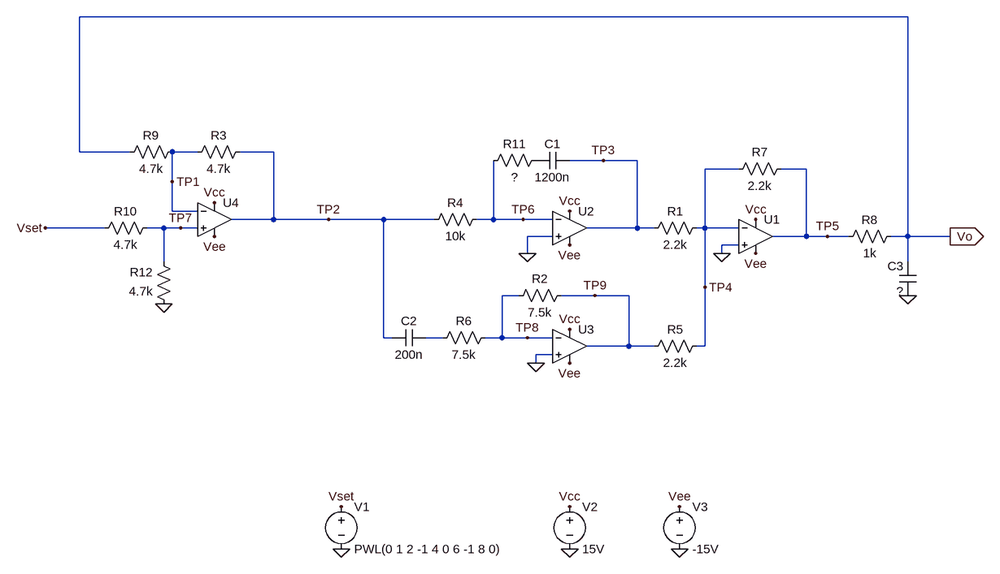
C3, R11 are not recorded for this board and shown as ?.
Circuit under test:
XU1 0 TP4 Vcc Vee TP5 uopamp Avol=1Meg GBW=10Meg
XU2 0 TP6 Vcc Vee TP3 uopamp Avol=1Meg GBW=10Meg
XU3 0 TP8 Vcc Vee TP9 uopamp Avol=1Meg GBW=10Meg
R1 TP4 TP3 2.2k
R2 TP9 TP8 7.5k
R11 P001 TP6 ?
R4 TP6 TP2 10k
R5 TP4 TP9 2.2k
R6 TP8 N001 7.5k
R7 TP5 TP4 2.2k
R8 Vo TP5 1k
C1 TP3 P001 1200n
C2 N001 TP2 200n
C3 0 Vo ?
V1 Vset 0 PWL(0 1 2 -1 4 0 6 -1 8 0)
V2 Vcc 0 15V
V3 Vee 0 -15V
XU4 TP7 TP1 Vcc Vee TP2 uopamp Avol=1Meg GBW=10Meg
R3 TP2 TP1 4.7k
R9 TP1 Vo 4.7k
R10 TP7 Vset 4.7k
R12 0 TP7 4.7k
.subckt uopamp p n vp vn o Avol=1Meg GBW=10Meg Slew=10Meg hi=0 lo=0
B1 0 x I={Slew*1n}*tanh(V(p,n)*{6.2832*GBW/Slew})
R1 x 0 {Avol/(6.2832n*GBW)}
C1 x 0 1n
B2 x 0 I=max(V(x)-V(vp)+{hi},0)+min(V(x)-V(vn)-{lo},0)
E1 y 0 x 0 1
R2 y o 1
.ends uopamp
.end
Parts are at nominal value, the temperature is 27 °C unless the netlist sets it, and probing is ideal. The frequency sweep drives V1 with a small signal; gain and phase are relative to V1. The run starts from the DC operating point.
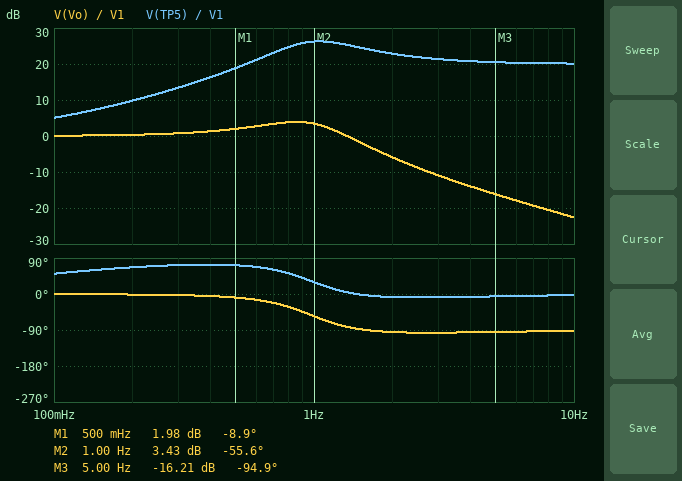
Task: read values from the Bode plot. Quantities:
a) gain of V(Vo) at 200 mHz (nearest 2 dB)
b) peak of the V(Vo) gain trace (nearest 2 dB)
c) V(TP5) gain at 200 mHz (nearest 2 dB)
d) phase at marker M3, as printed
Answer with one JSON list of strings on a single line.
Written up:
["0 dB", "4 dB", "10 dB", "-94.9 deg"]
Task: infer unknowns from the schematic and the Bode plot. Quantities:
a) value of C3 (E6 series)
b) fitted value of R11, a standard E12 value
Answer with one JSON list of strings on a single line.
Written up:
["2.2 mF", "100 kΩ"]
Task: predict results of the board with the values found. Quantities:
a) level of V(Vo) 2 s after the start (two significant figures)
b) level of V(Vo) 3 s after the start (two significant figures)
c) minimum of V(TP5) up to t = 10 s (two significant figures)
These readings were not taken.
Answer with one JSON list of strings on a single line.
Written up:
["-990 mV", "-490 mV", "-3.3 V"]
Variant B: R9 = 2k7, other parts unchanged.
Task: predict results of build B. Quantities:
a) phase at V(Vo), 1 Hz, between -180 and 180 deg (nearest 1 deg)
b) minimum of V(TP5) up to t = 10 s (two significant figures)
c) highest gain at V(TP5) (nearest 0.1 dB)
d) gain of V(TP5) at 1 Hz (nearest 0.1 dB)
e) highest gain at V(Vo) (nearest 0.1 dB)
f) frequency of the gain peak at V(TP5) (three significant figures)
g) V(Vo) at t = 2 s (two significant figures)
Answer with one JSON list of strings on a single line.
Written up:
["-26 deg", "-2.6 V", "25.8 dB", "23.6 dB", "0.8 dB", "1.53 Hz", "-780 mV"]
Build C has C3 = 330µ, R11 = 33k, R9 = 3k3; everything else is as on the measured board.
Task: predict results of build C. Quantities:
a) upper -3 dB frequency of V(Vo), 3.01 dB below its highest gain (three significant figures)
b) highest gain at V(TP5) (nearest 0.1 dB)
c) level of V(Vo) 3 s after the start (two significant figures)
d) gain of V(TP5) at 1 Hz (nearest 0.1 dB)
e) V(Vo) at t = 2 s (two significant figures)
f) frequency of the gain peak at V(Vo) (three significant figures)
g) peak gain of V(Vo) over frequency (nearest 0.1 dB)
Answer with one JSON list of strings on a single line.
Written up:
["3.94 Hz", "17.0 dB", "-430 mV", "6.8 dB", "-840 mV", "2.51 Hz", "1.5 dB"]
